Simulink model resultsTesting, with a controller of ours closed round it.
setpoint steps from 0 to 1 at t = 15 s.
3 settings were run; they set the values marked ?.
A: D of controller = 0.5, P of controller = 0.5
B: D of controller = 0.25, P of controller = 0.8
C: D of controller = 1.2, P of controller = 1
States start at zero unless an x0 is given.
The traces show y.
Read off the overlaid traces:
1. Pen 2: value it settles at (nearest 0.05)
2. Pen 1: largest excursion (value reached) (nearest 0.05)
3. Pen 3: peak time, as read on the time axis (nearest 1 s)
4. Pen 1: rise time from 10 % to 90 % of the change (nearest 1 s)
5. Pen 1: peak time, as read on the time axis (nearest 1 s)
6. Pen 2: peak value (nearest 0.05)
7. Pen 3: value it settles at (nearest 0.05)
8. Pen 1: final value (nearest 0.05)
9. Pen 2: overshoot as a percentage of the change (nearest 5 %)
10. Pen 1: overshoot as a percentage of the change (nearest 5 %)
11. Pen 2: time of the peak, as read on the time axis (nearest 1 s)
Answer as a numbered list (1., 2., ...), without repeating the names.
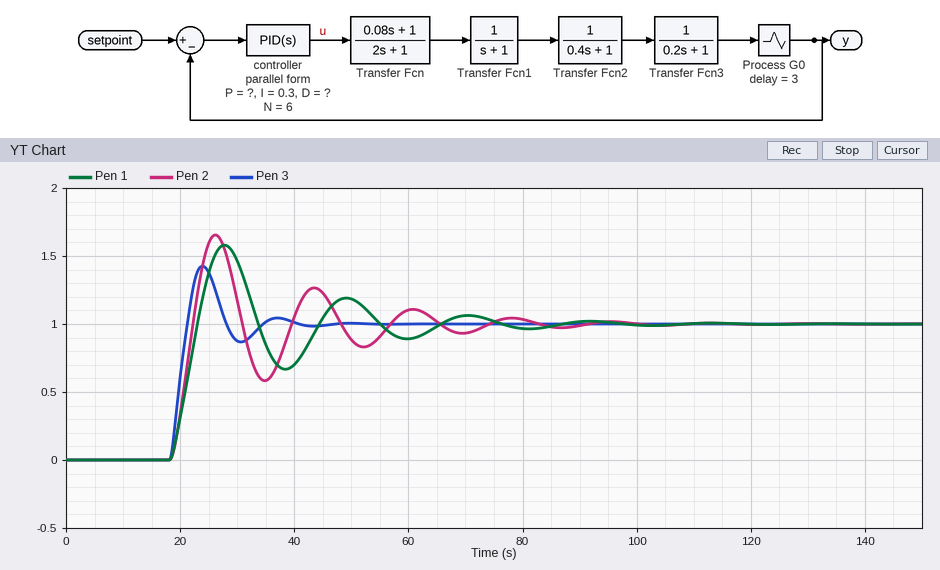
1. 1.00
2. 1.60
3. 24 s
4. 4 s
5. 28 s
6. 1.65
7. 1.00
8. 1.00
9. 65 %
10. 60 %
11. 26 s
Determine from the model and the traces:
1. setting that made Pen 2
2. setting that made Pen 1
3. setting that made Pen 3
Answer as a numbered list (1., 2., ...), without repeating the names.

1. B
2. A
3. C
